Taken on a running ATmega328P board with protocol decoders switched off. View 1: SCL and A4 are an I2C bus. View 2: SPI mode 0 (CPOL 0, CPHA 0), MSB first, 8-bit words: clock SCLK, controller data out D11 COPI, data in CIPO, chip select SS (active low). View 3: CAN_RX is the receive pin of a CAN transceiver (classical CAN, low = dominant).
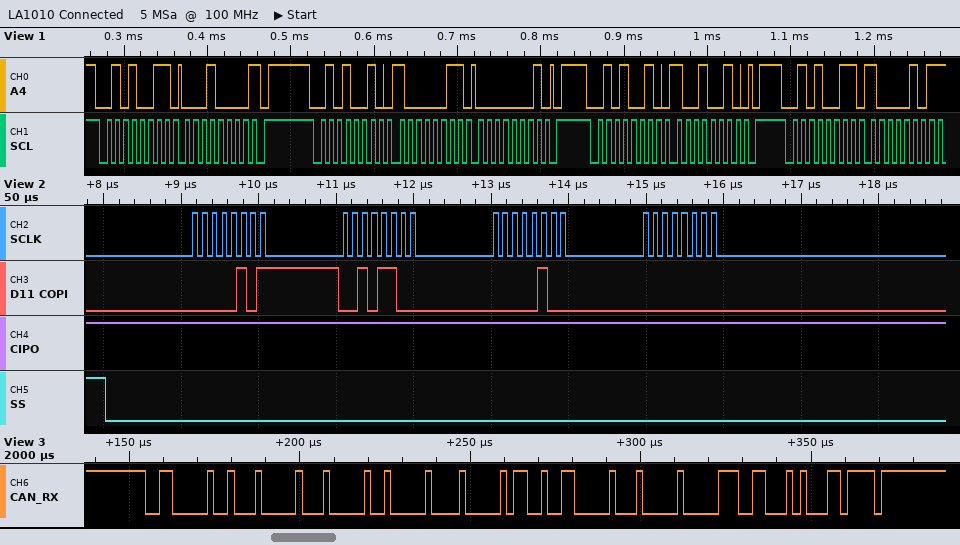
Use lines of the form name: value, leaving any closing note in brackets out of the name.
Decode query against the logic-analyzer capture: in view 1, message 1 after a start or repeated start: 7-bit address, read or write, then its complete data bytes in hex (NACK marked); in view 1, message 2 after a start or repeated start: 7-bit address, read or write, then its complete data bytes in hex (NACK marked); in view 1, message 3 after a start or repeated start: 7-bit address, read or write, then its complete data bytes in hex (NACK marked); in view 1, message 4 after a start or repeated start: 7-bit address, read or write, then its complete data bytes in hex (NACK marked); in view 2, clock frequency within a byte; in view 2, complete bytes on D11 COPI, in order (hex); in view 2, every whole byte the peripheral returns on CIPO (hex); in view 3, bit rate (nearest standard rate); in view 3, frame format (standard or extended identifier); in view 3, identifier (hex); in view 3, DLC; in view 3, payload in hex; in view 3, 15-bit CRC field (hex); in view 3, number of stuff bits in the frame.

in view 1, message 1 after a start or repeated start: 7-bit address, read or write, then its complete data bytes in hex: 0x29 read: 10 NACK
in view 1, message 2 after a start or repeated start: 7-bit address, read or write, then its complete data bytes in hex: 0x29 write: 83 01
in view 1, message 3 after a start or repeated start: 7-bit address, read or write, then its complete data bytes in hex: 0x29 write: 92
in view 1, message 4 after a start or repeated start: 7-bit address, read or write, then its complete data bytes in hex: 0x29 read: 85 NACK
in view 2, clock frequency within a byte: 8 MHz
in view 2, complete bytes on D11 COPI, in order: 0x05 0x2C 0x04 0x00
in view 2, every whole byte the peripheral returns on CIPO: 0xFF 0xFF 0xFF 0xFF
in view 3, bit rate: 500 kbit/s
in view 3, frame format: standard
in view 3, identifier: 0x301
in view 3, DLC: 8
in view 3, payload in hex: 04 04 01 03 26 01 00 33
in view 3, 15-bit CRC field: 0x0A37
in view 3, number of stuff bits in the frame: 8
